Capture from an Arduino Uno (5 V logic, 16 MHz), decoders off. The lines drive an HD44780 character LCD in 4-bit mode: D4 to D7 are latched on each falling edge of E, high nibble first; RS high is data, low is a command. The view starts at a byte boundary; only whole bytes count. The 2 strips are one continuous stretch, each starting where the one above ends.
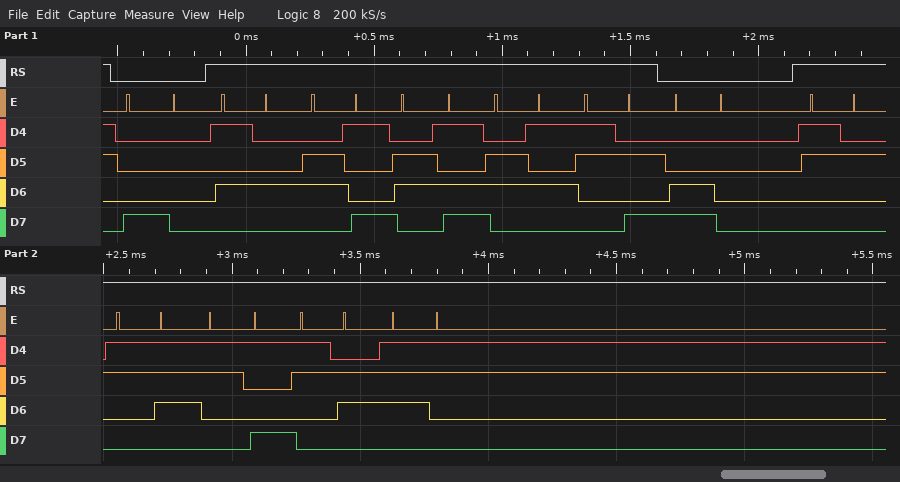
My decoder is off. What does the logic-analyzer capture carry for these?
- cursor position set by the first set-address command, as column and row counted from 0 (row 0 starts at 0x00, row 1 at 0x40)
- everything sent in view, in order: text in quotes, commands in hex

column 0, row 0
0x80 "Time:" 0xC0 "2796s"
